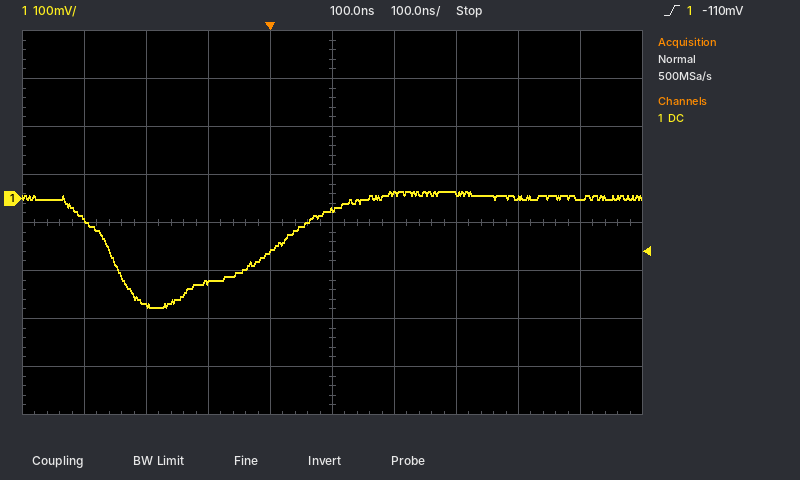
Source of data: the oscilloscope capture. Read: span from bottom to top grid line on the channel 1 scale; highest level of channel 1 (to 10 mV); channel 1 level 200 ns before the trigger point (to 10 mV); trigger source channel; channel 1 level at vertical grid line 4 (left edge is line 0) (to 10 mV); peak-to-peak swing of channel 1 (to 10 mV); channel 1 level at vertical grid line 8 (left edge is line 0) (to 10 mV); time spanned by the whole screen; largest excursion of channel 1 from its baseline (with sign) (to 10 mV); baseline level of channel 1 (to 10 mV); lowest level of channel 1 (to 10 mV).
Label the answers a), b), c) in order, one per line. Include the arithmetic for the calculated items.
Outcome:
a) 800 mV
b) 10 mV
c) -220 mV
d) channel 1
e) -110 mV
f) 10 mV − (-230 mV) = 240 mV
g) 0 mV
h) 1 µs
i) -230 mV − (0 mV) = -230 mV
j) 0 mV
k) -230 mV
